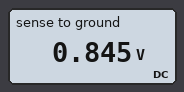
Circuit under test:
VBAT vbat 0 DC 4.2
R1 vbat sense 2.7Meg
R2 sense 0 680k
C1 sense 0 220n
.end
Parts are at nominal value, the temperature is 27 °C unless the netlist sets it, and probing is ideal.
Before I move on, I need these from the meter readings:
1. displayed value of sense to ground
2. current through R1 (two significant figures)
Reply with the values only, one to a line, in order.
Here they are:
0.845 V
1.2 µA
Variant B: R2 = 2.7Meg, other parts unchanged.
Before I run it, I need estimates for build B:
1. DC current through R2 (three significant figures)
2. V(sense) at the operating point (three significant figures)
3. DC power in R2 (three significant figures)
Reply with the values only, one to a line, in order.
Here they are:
778 nA
2.10 V
1.63 µW
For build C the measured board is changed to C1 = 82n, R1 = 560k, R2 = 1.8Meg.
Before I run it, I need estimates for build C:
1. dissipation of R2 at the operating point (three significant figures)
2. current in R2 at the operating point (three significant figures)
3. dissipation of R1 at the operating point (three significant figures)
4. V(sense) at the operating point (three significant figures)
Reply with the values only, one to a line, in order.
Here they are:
5.70 µW
1.78 µA
1.77 µW
3.20 V
